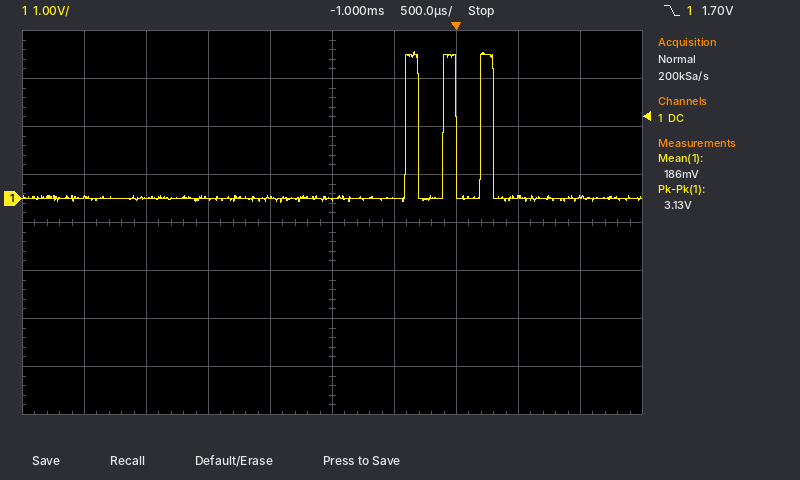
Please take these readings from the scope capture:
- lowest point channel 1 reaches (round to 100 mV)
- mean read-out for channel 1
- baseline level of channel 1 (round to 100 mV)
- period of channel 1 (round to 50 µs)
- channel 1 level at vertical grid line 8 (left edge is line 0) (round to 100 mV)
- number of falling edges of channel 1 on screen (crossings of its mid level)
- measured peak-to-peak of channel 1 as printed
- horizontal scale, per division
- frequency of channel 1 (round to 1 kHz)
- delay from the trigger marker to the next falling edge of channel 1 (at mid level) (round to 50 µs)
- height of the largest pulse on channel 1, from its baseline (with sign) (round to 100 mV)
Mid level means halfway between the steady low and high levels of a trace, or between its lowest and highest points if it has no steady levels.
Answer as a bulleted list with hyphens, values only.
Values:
- -100 mV
- 186 mV
- 0.0 V
- 300 µs
- 0.0 V
- 3
- 3.13 V
- 500 µs
- 3 kHz
- 300 µs
- +3.1 V
